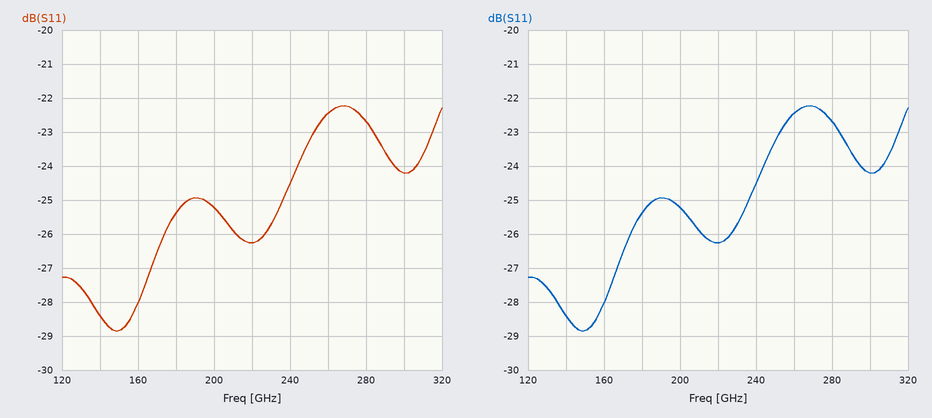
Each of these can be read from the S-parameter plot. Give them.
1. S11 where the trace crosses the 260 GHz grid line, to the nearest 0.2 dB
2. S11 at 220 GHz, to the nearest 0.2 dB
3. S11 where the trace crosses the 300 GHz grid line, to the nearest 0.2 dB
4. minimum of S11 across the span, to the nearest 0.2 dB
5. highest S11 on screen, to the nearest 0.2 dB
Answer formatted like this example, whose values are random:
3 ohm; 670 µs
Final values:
-22.4 dB; -26.2 dB; -24.2 dB; -28.8 dB; -22.2 dB
